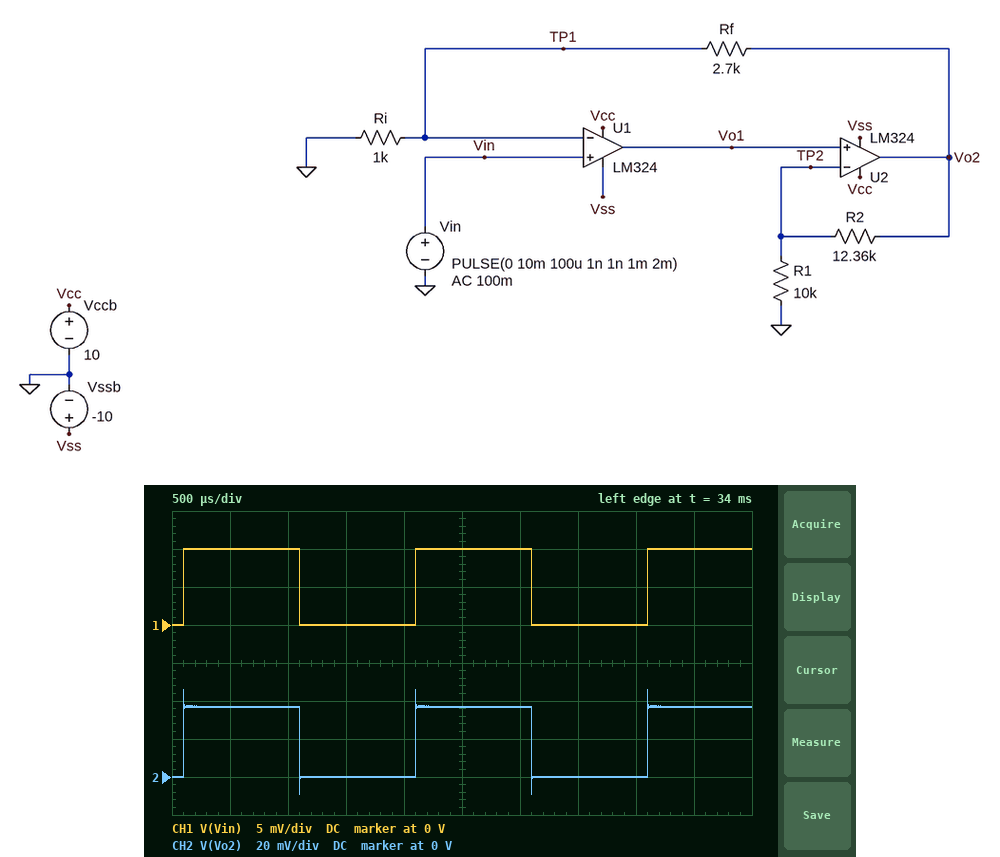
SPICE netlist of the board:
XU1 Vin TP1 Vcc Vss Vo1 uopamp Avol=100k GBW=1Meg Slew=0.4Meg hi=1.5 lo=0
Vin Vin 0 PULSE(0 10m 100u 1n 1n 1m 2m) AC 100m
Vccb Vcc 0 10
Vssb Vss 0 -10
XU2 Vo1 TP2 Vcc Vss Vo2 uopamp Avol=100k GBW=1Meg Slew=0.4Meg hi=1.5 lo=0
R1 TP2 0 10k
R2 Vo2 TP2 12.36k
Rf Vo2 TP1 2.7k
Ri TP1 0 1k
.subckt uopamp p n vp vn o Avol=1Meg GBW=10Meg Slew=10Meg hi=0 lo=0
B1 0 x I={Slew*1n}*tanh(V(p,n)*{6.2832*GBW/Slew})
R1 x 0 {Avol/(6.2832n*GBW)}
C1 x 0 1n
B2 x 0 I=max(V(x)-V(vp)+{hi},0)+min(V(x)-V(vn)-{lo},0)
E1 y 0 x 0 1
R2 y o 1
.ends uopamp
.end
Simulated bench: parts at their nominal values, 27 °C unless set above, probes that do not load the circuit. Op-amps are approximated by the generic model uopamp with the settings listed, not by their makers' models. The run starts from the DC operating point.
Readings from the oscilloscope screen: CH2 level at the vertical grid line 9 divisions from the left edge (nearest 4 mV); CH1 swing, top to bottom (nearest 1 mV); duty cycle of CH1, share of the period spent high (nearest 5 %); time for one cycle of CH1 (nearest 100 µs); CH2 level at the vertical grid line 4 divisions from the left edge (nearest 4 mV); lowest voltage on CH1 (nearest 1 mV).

36 mV
10 mV
50 %
2.0 ms
0 V
0 V
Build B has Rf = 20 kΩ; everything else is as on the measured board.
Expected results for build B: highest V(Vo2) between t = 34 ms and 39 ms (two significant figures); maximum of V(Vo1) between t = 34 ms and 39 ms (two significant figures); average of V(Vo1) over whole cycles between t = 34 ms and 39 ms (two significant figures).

210 mV
94 mV
47 mV
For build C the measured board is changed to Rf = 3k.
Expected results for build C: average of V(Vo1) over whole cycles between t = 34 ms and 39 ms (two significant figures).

8.9 mV
